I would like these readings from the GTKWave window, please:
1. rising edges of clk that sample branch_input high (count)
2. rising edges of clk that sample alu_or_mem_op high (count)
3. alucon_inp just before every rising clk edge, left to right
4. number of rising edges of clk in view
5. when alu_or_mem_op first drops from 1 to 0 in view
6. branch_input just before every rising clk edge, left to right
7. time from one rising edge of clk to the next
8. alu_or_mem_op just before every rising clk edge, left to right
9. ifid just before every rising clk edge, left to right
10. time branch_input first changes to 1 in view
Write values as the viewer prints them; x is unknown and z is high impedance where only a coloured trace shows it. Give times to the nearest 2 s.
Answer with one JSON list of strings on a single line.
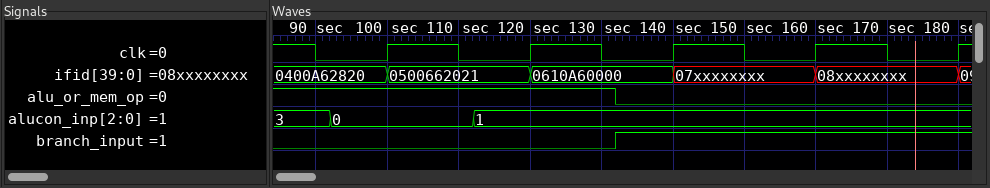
["3", "2", "0, 1, 1, 1, 1", "5", "132 s", "0 0 1 1 1", "20 s", "1 1 0 0 0", "0400A62820, 0500662021, 0610A60000, 07xxxxxxxx, 08xxxxxxxx", "132 s"]
